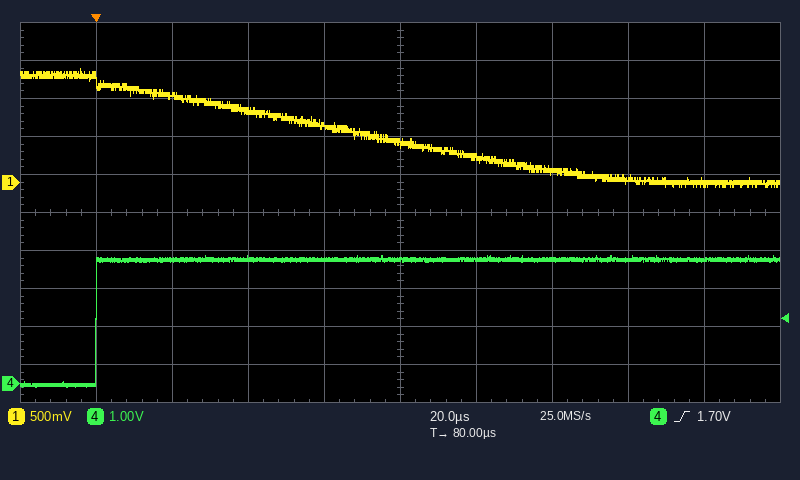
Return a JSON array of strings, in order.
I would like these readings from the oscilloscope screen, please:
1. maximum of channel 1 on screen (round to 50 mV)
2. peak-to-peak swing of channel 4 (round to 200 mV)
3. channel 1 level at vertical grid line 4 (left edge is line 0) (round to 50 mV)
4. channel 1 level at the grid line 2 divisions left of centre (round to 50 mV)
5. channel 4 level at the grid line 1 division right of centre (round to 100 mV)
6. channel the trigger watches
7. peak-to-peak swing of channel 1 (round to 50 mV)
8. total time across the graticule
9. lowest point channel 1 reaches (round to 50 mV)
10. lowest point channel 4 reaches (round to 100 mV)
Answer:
["1.50 V", "3.4 V", "750 mV", "950 mV", "3.3 V", "channel 4", "1.55 V", "200 µs", "-50 mV", "-100 mV"]
